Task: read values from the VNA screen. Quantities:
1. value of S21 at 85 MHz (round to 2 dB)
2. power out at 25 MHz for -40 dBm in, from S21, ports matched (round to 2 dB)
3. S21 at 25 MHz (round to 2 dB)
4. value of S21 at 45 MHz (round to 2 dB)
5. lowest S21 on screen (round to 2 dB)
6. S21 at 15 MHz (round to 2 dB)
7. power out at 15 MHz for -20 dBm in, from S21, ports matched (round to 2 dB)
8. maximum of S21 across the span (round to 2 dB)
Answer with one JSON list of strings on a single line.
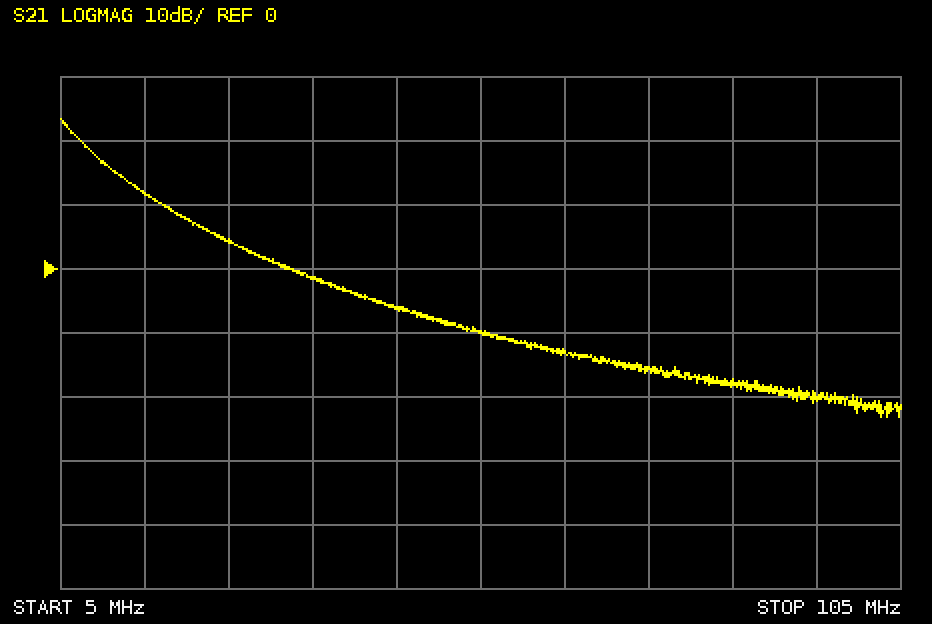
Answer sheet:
["-18 dB", "-36 dBm", "4 dB", "-6 dB", "-24 dB", "12 dB", "-8 dBm", "24 dB"]
